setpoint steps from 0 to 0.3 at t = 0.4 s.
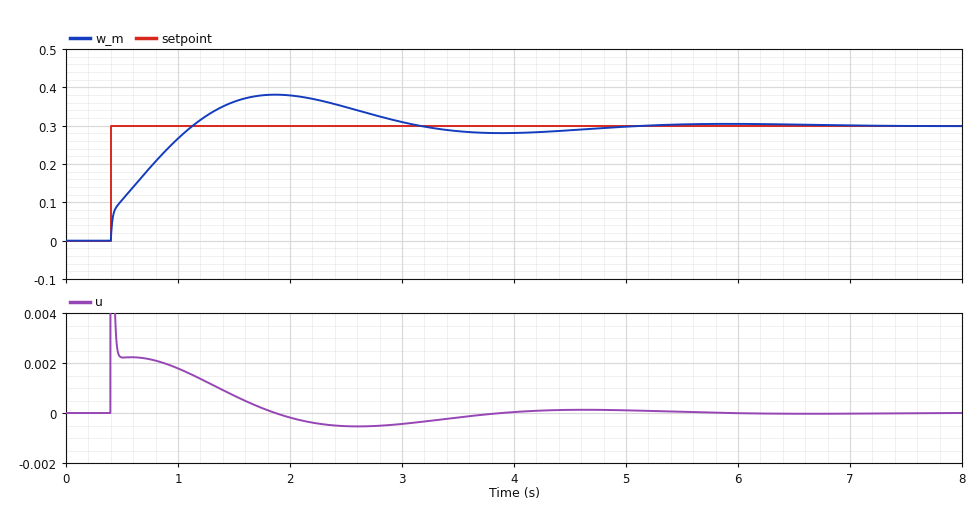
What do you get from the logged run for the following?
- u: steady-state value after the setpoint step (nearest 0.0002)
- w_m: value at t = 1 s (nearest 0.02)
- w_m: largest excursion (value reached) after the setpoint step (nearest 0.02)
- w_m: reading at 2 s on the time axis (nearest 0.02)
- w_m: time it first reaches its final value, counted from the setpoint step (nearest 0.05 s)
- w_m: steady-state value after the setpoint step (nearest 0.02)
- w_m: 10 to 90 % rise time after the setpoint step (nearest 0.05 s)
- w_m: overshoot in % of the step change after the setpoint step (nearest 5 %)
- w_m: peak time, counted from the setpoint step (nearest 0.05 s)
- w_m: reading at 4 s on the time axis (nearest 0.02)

0.0000
0.26
0.38
0.38
0.75 s
0.30
0.60 s
25 %
1.45 s
0.28
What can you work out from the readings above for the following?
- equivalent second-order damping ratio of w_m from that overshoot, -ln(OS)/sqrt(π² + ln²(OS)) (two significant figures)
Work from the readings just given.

0.40
